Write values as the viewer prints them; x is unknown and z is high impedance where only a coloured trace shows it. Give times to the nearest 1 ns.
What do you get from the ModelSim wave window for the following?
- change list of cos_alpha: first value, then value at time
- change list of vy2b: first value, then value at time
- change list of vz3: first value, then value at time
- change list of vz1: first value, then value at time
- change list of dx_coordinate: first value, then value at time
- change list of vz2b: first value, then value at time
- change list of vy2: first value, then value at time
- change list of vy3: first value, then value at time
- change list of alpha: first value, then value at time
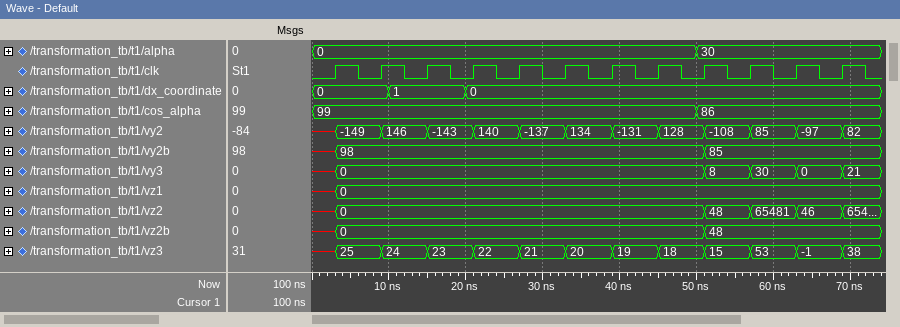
99, 86 at 50 ns
x, 98 at 3 ns, 85 at 51 ns
x, 25 at 3 ns, 24 at 9 ns, 23 at 15 ns, 22 at 21 ns, 21 at 27 ns, 20 at 33 ns, 19 at 39 ns, 18 at 45 ns, 15 at 51 ns, 53 at 57 ns, -1 at 63 ns, 38 at 69 ns
x, 0 at 3 ns
0, 1 at 10 ns, 0 at 20 ns
x, 0 at 3 ns, 48 at 51 ns
x, -149 at 3 ns, 146 at 9 ns, -143 at 15 ns, 140 at 21 ns, -137 at 27 ns, 134 at 33 ns, -131 at 39 ns, 128 at 45 ns, -108 at 51 ns, 85 at 57 ns, -97 at 63 ns, 82 at 69 ns
x, 0 at 3 ns, 8 at 51 ns, 30 at 57 ns, 0 at 63 ns, 21 at 69 ns
0, 30 at 50 ns
